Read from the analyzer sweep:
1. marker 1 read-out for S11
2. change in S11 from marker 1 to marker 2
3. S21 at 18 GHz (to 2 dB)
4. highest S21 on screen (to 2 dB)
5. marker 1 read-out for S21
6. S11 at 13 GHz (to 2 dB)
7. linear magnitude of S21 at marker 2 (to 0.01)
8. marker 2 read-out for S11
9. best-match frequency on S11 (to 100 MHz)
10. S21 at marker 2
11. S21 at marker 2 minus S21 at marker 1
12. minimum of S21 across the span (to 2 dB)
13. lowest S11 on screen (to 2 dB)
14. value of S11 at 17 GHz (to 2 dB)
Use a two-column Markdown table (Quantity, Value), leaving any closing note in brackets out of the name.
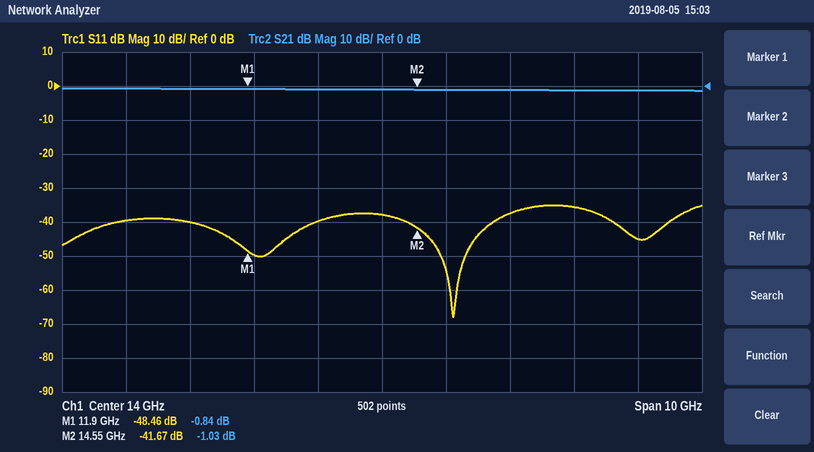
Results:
| Quantity | Value |
|---|---|
| marker 1 read-out for S11 | -48.46 dB |
| change in S11 from marker 1 to marker 2 | 6.79 dB |
| S21 at 18 GHz | -2 dB |
| highest S21 on screen | 0 dB |
| marker 1 read-out for S21 | -0.84 dB |
| S11 at 13 GHz | -40 dB |
| linear magnitude of S21 at marker 2 | 0.89 |
| marker 2 read-out for S11 | -41.67 dB |
| best-match frequency on S11 | 15.1 GHz |
| S21 at marker 2 | -1.03 dB |
| S21 at marker 2 minus S21 at marker 1 | -0.19 dB |
| minimum of S21 across the span | -2 dB |
| lowest S11 on screen | -68 dB |
| value of S11 at 17 GHz | -36 dB |
